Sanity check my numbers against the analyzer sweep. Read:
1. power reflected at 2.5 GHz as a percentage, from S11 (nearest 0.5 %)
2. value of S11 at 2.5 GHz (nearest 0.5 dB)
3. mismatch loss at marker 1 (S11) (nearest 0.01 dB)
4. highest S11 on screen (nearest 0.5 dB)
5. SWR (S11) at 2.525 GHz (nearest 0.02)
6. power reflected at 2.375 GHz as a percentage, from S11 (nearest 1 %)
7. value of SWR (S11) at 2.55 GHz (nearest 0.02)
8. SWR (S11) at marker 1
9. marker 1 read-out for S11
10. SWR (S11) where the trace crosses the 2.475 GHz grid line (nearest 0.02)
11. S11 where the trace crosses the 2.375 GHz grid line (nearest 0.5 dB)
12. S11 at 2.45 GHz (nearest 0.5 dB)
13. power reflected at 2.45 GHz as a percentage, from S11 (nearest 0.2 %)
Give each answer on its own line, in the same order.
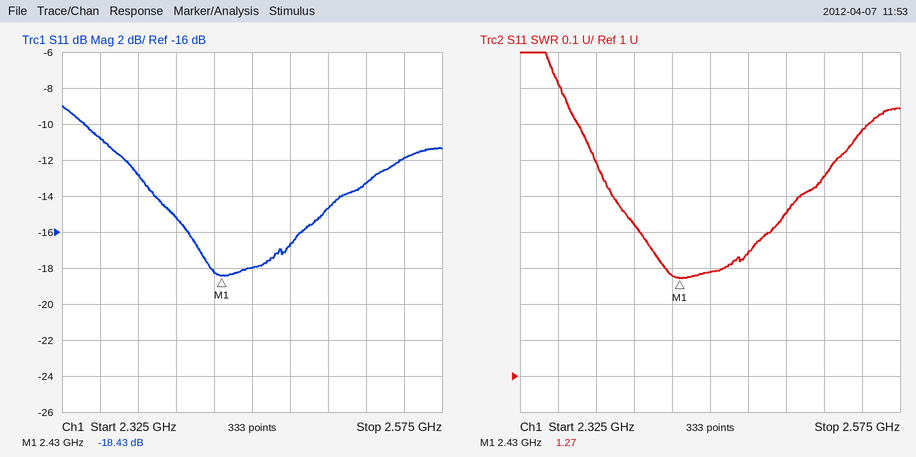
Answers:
3.5 %
-14.5 dB
0.06 dB
-9.0 dB
1.56
5 %
1.68
1.27
-18.43 dB
1.34
-13.0 dB
-18.0 dB
1.6 %
